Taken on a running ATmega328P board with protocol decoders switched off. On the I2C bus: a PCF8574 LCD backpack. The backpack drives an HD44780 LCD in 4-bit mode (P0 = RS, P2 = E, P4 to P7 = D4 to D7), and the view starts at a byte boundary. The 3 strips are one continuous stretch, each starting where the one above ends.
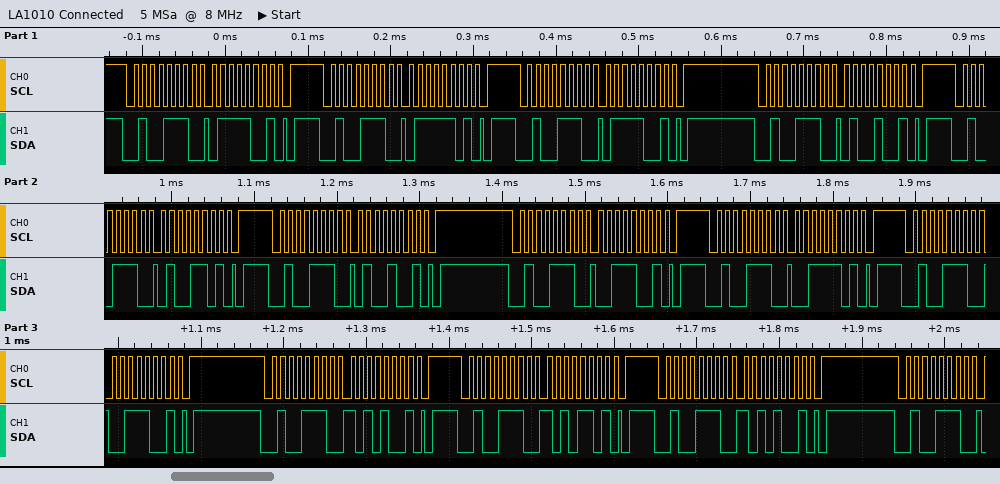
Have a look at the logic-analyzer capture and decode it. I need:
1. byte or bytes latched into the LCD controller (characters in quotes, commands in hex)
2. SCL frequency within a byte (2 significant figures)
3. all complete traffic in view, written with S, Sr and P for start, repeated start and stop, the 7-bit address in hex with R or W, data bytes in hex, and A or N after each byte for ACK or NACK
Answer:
't' ':'
100 kHz
S 27W A 79 A P S 27W A 7D A P S 27W A 79 A P S 27W A 49 A P S 27W A 4D A P S 27W A 49 A P S 27W A 39 A P S 27W A 3D A P S 27W A 39 A P S 27W A A9 A P S 27W A AD A P S 27W A A9 A P S 27W A
